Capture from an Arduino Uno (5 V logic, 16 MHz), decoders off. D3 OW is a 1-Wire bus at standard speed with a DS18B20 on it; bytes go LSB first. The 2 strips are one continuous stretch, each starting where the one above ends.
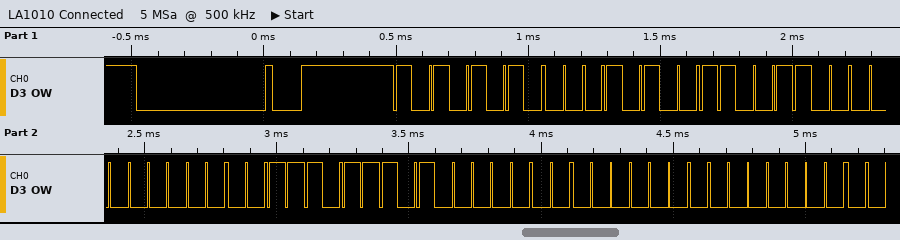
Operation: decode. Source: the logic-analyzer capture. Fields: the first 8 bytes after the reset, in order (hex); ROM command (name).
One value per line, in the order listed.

55 28 33 00 DC 05 00 00
Match ROM
